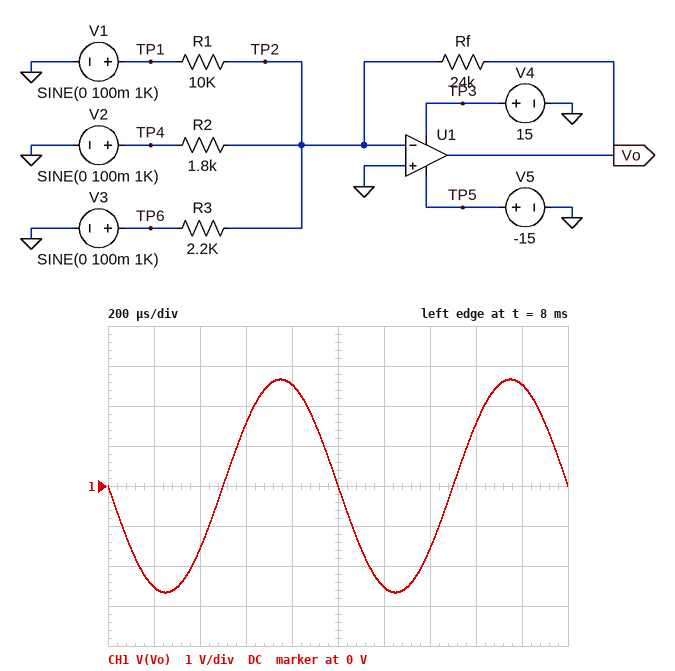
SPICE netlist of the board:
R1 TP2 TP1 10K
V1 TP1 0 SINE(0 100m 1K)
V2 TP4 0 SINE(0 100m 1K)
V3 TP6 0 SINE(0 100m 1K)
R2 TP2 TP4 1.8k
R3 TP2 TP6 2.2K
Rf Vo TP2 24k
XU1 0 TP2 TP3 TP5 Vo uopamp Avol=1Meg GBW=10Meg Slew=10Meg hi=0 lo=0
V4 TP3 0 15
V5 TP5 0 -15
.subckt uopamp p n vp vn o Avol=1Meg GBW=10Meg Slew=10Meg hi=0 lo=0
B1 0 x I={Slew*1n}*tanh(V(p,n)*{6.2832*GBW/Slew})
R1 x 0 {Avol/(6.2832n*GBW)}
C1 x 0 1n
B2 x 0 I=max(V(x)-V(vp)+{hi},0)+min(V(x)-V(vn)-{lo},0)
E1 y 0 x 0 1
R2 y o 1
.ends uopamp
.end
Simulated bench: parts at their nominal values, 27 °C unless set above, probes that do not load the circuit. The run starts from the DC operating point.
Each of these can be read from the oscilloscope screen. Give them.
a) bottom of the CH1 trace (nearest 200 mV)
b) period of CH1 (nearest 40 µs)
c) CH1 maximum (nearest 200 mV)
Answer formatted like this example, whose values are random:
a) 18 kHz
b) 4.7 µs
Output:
a) -2.6 V
b) 1.00 ms
c) 2.6 V
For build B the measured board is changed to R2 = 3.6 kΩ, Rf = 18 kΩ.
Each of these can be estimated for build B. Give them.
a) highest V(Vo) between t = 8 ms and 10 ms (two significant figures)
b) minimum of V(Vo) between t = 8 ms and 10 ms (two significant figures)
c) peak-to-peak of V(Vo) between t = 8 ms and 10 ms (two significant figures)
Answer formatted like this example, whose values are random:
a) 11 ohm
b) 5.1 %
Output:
a) 1.5 V
b) -1.5 V
c) 3.0 V
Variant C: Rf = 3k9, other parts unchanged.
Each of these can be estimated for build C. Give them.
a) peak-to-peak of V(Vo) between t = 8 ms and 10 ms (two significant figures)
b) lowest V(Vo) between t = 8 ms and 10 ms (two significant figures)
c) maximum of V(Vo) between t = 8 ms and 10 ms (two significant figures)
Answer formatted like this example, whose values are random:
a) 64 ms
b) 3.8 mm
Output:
a) 870 mV
b) -430 mV
c) 430 mV
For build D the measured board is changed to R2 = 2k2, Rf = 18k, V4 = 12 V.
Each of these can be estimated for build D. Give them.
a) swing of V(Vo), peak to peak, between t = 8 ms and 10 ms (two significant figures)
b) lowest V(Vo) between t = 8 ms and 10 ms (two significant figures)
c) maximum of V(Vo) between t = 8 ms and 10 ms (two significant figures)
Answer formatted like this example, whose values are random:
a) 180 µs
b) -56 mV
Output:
a) 3.6 V
b) -1.8 V
c) 1.8 V
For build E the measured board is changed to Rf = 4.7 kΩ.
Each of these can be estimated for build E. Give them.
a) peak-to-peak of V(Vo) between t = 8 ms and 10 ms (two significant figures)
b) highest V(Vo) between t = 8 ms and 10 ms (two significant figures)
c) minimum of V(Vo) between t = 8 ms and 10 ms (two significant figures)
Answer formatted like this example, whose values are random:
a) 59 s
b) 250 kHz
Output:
a) 1.0 V
b) 520 mV
c) -520 mV
